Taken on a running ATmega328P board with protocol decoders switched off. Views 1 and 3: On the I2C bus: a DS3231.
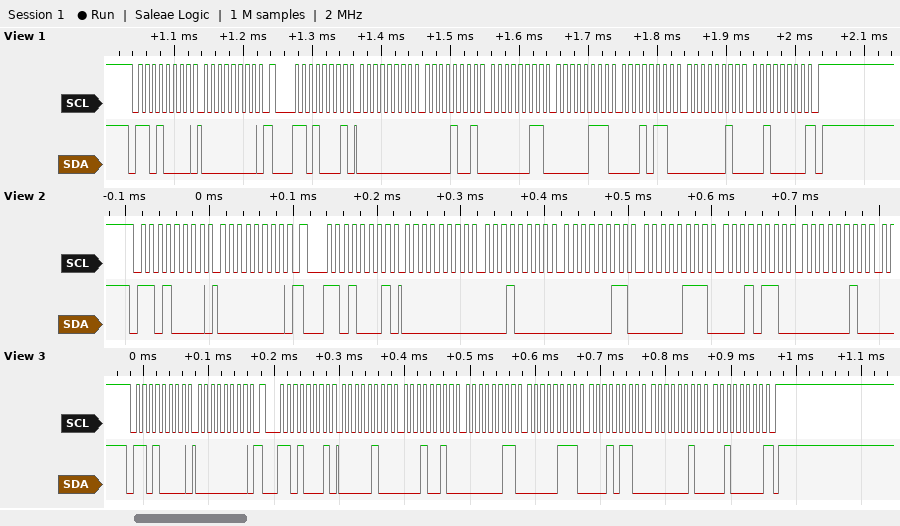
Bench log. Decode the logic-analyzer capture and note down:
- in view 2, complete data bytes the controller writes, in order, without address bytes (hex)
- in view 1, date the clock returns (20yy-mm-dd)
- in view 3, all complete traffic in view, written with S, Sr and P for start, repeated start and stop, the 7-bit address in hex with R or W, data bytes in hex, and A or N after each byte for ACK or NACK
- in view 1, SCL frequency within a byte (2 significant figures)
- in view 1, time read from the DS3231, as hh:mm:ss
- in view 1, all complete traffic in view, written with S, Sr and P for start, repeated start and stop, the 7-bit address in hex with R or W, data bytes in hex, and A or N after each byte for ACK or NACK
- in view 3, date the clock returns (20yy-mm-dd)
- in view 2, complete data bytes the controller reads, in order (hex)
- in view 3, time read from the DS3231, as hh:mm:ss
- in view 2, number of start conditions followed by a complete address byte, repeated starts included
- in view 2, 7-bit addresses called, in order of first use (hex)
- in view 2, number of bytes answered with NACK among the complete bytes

00
2020-02-16
S 68W A 00 A Sr 68R A 04 A 12 A 03 A 07 A 16 A 02 A 20 N P
100 kHz
03:09:00
S 68W A 00 A Sr 68R A 00 A 09 A 03 A 07 A 16 A 02 A 20 N P
2020-02-16
00 10 03 07 16 02
03:12:04
2
0x68
0
